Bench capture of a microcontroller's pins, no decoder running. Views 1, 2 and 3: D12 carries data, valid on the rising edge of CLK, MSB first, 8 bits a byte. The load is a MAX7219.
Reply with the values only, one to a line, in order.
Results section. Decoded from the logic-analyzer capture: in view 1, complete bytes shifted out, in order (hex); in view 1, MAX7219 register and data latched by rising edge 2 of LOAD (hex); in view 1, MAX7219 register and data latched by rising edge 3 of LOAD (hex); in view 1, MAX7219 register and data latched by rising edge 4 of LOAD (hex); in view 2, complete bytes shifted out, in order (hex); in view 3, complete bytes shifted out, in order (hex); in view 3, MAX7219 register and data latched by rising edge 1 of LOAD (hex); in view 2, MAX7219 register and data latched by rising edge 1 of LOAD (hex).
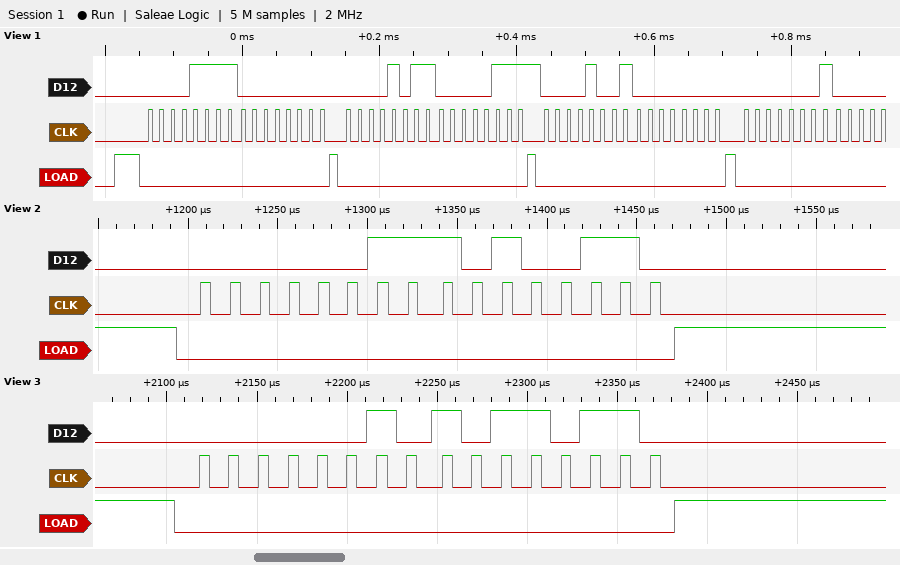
0F 00 0B 07 09 00 01
register 0xF, data 0x00
register 0xB, data 0x07
register 0x9, data 0x00
0x03 0xA6
02 B6
register 0x2, data 0xB6
register 0x3, data 0xA6
